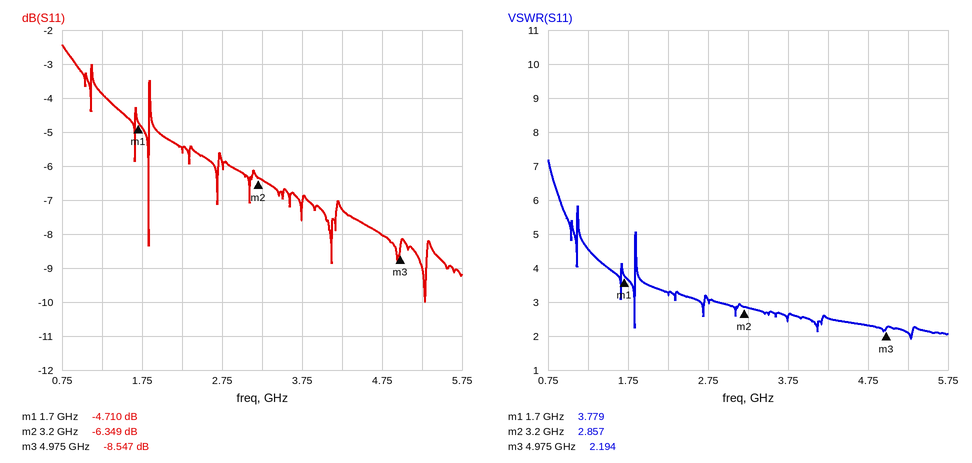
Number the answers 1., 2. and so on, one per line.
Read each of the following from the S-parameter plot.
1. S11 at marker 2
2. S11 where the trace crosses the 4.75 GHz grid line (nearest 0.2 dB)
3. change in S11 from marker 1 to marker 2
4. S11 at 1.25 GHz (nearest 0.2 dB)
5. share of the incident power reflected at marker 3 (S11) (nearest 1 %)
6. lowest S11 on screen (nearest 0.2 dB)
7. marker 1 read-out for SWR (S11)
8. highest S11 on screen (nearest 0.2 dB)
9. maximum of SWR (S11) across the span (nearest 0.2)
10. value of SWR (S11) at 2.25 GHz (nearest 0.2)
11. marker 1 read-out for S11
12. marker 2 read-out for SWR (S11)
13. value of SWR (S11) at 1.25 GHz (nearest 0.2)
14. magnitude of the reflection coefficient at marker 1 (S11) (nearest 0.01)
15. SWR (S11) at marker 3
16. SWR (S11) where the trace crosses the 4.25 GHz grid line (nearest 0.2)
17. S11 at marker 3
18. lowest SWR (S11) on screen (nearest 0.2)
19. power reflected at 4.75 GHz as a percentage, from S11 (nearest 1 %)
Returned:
1. -6.349 dB
2. -8.0 dB
3. -1.639 dB
4. -3.8 dB
5. 14 %
6. -10.0 dB
7. 3.779
8. -2.4 dB
9. 7.2
10. 3.2
11. -4.710 dB
12. 2.857
13. 4.6
14. 0.58
15. 2.194
16. 2.6
17. -8.547 dB
18. 2.0
19. 16 %
